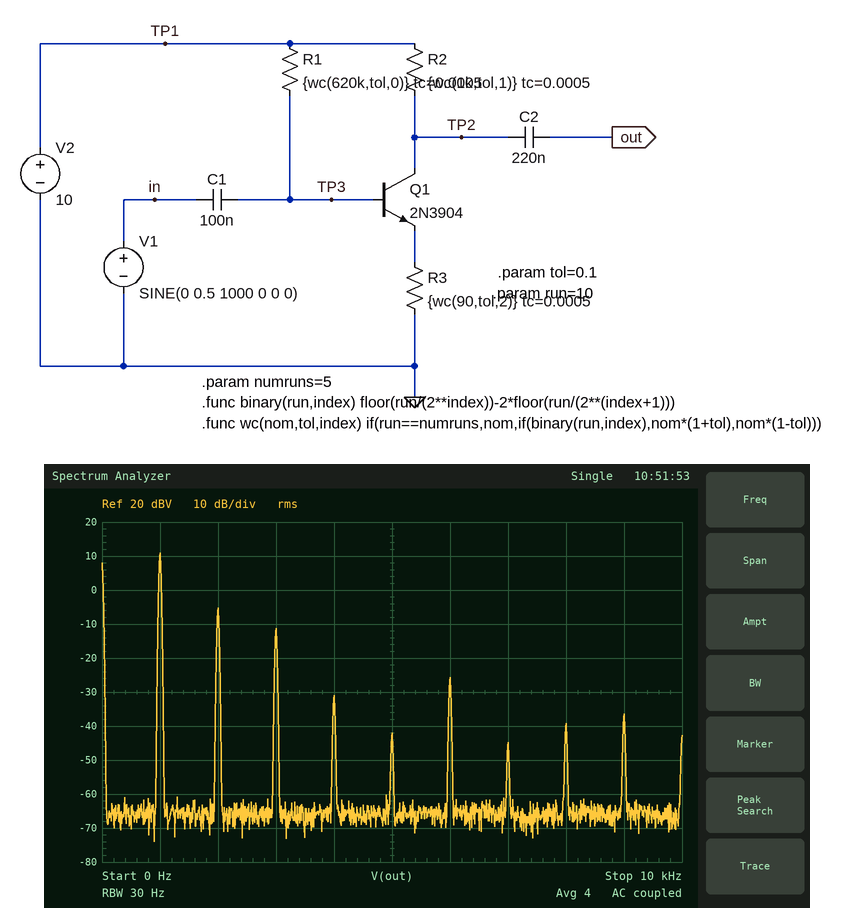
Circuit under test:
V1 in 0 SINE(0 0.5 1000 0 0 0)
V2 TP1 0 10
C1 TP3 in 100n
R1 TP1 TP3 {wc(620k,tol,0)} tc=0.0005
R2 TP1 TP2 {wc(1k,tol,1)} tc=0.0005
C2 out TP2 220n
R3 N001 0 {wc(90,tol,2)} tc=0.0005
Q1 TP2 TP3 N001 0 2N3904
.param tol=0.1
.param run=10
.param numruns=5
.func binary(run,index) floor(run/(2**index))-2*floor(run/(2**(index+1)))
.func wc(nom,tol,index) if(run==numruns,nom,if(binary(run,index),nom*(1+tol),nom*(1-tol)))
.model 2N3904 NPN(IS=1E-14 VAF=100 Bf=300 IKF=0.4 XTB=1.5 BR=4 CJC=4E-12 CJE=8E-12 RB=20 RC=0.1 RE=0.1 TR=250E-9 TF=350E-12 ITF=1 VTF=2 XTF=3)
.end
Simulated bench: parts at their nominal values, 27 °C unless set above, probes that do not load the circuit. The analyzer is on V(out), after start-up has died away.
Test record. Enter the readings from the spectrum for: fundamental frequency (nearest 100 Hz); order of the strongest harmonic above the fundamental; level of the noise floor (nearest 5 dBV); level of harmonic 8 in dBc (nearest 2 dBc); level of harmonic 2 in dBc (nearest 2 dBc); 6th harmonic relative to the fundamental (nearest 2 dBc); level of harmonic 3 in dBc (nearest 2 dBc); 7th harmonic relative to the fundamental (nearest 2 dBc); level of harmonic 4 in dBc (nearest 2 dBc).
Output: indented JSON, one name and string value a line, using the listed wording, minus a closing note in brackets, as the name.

{
  "fundamental frequency": "1.0 kHz",
  "order of the strongest harmonic above the fundamental": "2",
  "level of the noise floor": "-65 dBV",
  "level of harmonic 8 in dBc": "-50 dBc",
  "level of harmonic 2 in dBc": "-16 dBc",
  "6th harmonic relative to the fundamental": "-36 dBc",
  "level of harmonic 3 in dBc": "-22 dBc",
  "7th harmonic relative to the fundamental": "-56 dBc",
  "level of harmonic 4 in dBc": "-42 dBc"
}
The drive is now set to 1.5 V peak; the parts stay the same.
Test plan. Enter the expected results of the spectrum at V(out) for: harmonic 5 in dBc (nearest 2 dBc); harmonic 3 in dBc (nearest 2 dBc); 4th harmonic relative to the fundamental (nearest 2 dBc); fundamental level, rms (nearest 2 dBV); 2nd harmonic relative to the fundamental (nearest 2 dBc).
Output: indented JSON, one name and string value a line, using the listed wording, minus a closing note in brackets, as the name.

{
  "harmonic 5 in dBc": "-20 dBc",
  "harmonic 3 in dBc": "-10 dBc",
  "4th harmonic relative to the fundamental": "-30 dBc",
  "fundamental level, rms": "8 dBV",
  "2nd harmonic relative to the fundamental": "-4 dBc"
}
